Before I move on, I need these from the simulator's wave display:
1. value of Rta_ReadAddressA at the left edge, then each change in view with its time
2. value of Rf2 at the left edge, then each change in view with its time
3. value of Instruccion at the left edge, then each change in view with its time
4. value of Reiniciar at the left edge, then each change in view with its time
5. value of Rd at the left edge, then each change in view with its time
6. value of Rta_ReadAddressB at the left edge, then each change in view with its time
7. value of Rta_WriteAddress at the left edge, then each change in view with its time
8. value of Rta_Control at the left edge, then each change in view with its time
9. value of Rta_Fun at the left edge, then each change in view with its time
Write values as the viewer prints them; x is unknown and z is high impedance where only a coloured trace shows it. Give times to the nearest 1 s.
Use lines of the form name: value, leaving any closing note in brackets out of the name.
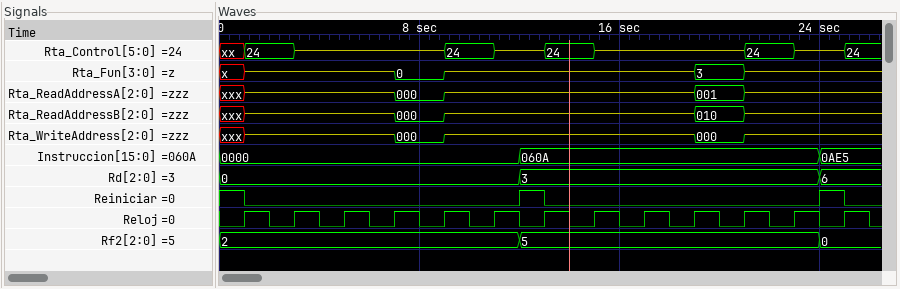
value of Rta_ReadAddressA at the left edge, then each change in view with its time: xxx, z at 1 s, 000 at 7 s, z at 9 s, 001 at 19 s, z at 21 s
value of Rf2 at the left edge, then each change in view with its time: 2, 5 at 12 s, 0 at 24 s
value of Instruccion at the left edge, then each change in view with its time: 0000, 060A at 12 s, 0AE5 at 24 s
value of Reiniciar at the left edge, then each change in view with its time: 1, 0 at 1 s, 1 at 12 s, 0 at 13 s, 1 at 24 s, 0 at 25 s
value of Rd at the left edge, then each change in view with its time: 0, 3 at 12 s, 6 at 24 s
value of Rta_ReadAddressB at the left edge, then each change in view with its time: xxx, z at 1 s, 000 at 7 s, z at 9 s, 010 at 19 s, z at 21 s
value of Rta_WriteAddress at the left edge, then each change in view with its time: xxx, z at 1 s, 000 at 7 s, z at 9 s, 000 at 19 s, z at 21 s
value of Rta_Control at the left edge, then each change in view with its time: xx, 24 at 1 s, z at 3 s, 24 at 9 s, z at 11 s, 24 at 13 s, z at 15 s, 24 at 21 s, z at 23 s, 24 at 25 s
value of Rta_Fun at the left edge, then each change in view with its time: x, z at 1 s, 0 at 7 s, z at 9 s, 3 at 19 s, z at 21 s
